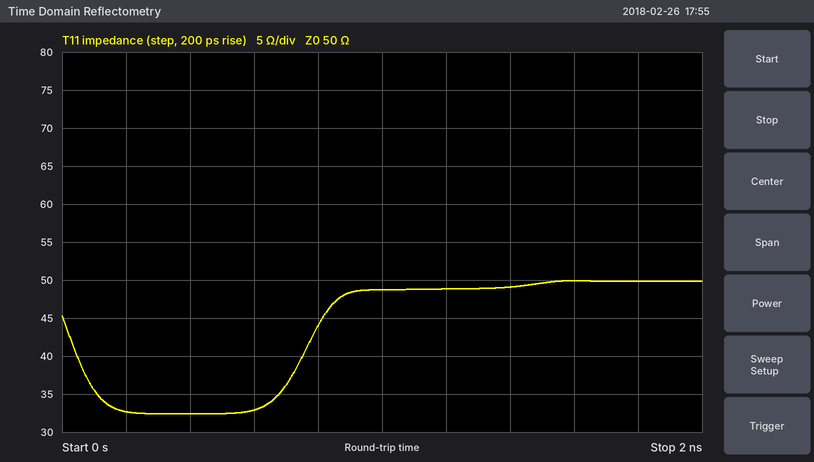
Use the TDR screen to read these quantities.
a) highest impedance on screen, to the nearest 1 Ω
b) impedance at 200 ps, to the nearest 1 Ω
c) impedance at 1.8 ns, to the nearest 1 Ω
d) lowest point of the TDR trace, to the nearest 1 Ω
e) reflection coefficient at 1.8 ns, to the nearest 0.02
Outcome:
50 Ω
33 Ω
50 Ω
32 Ω
0.00
